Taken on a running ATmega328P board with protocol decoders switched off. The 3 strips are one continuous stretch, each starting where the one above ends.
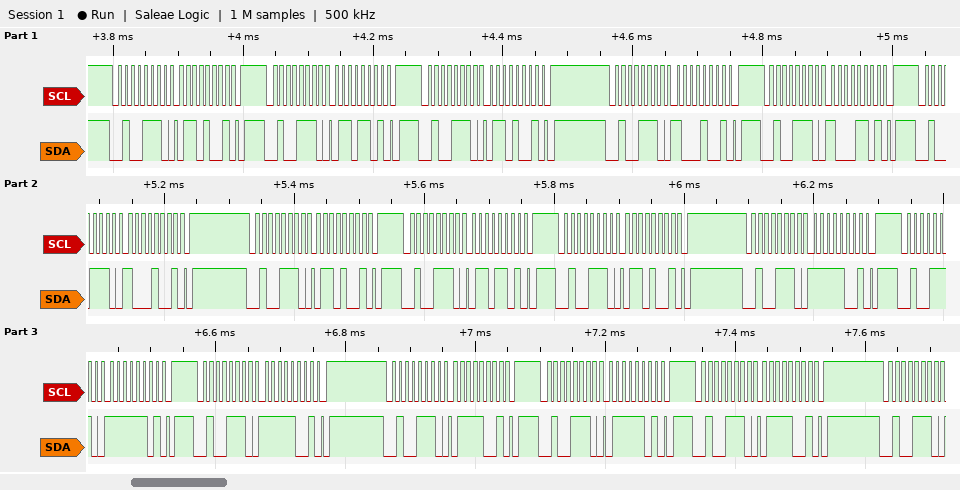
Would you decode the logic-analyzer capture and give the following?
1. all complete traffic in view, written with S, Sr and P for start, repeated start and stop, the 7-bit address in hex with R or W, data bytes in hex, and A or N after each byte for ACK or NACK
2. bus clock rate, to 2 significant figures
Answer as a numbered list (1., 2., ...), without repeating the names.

1. S 27W A 69 A P S 27W A 6D A P S 27W A 69 A P S 27W A 89 A P S 27W A 8D A P S 27W A 89 A P S 27W A 69 A P S 27W A 6D A P S 27W A 69 A P S 27W A F9 A P S 27W A FD A P S 27W A F9 A P S 27W A 79 A P S 27W A 7D A P S 27W A 79 A P S 27W A
2. 100 kHz
